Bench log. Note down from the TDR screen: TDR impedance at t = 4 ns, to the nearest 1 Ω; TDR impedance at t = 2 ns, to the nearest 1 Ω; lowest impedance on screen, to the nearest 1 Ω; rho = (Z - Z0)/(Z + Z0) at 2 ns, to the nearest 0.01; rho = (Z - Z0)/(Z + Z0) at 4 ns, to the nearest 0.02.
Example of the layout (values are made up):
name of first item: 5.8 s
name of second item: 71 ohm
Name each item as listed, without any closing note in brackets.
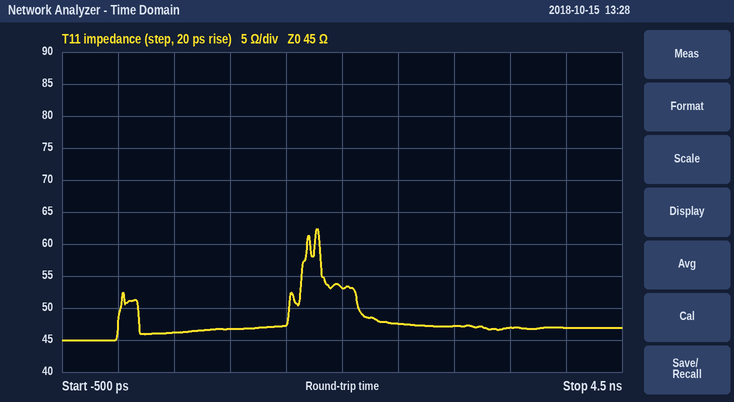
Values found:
TDR impedance at t = 4 ns, to the nearest 1 Ω: 47 Ω
TDR impedance at t = 2 ns, to the nearest 1 Ω: 53 Ω
lowest impedance on screen, to the nearest 1 Ω: 45 Ω
rho = (Z - Z0)/(Z + Z0) at 2 ns, to the nearest 0.01: +0.08
rho = (Z - Z0)/(Z + Z0) at 4 ns, to the nearest 0.02: +0.02
